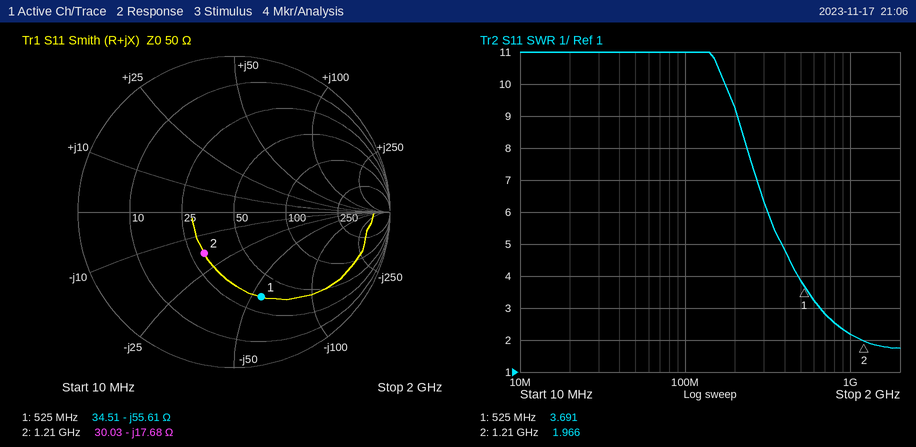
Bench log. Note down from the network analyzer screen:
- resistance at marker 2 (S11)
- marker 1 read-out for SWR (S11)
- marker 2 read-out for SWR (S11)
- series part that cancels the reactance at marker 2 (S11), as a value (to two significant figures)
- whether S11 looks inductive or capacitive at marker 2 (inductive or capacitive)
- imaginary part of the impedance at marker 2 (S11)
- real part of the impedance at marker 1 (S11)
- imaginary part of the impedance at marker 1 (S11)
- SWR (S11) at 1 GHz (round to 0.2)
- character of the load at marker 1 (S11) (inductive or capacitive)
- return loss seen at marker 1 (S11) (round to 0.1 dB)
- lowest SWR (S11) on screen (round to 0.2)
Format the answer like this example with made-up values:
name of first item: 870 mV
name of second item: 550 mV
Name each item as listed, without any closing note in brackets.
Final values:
resistance at marker 2: 30.03 Ω
marker 1 read-out for SWR: 3.691
marker 2 read-out for SWR: 1.966
series part that cancels the reactance at marker 2 (S11), as a value: 2.3 nH
whether S11 looks inductive or capacitive at marker 2: capacitive
imaginary part of the impedance at marker 2: -17.68 Ω
real part of the impedance at marker 1: 34.51 Ω
imaginary part of the impedance at marker 1: -55.61 Ω
SWR (S11) at 1 GHz: 2.2
character of the load at marker 1 (S11): capacitive
return loss seen at marker 1 (S11): 4.9 dB
lowest SWR (S11) on screen: 1.8
